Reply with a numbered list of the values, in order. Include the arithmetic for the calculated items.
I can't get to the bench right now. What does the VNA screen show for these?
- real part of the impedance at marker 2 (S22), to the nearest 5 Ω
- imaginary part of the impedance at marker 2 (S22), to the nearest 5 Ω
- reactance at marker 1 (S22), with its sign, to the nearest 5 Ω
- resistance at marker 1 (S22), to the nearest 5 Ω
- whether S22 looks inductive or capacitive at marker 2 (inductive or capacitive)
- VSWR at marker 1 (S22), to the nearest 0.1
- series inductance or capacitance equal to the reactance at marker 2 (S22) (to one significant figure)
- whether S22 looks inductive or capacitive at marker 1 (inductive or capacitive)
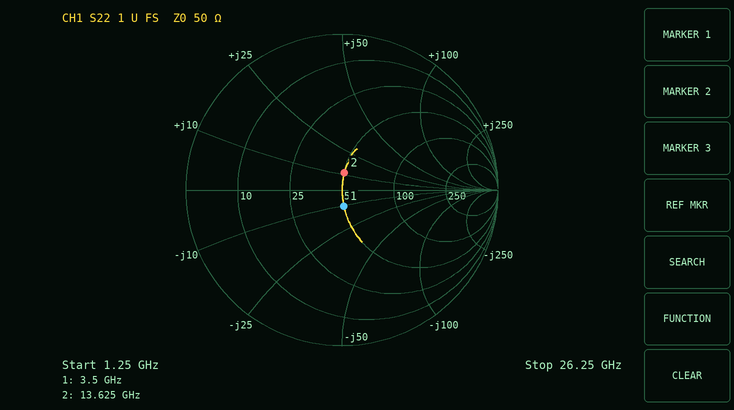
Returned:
1. 50 Ω
2. +10 Ω
3. -10 Ω
4. 50 Ω
5. inductive
6. 1.2
7. L = 10 Ω/(2π × 13.625 GHz) ≈ 117 pH, so 100 pH to one significant figure
8. capacitive
